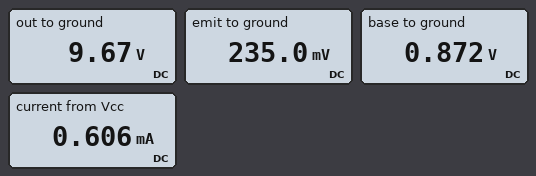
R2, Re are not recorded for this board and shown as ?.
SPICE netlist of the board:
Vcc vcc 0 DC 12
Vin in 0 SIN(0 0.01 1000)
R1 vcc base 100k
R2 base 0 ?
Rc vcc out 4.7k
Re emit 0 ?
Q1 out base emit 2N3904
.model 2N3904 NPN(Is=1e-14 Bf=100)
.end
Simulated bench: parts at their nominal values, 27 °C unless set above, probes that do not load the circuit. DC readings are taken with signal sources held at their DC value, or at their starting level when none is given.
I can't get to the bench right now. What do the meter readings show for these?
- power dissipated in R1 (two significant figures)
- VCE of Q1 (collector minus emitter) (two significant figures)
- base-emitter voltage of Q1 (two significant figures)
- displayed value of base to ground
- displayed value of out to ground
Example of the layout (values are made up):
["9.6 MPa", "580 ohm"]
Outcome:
["1.2 mW", "9.4 V", "640 mV", "0.872 V", "9.67 V"]
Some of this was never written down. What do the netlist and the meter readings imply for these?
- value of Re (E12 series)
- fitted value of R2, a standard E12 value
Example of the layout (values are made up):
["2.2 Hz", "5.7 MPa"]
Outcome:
["470 Ω", "8.2 kΩ"]
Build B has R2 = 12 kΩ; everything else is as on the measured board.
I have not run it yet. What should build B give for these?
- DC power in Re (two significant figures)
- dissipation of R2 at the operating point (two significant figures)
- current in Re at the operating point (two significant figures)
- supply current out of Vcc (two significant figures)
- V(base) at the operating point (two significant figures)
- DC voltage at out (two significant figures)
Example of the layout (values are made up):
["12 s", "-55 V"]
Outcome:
["560 µW", "110 µW", "1.1 mA", "1.2 mA", "1.2 V", "6.9 V"]
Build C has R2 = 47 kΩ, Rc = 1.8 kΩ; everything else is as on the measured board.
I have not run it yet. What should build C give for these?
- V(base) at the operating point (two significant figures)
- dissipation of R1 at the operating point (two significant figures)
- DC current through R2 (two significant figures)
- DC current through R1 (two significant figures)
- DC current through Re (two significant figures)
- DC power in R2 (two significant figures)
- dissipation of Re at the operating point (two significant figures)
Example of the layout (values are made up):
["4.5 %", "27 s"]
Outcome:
["2.6 V", "890 µW", "55 µA", "94 µA", "4.0 mA", "140 µW", "7.5 mW"]
